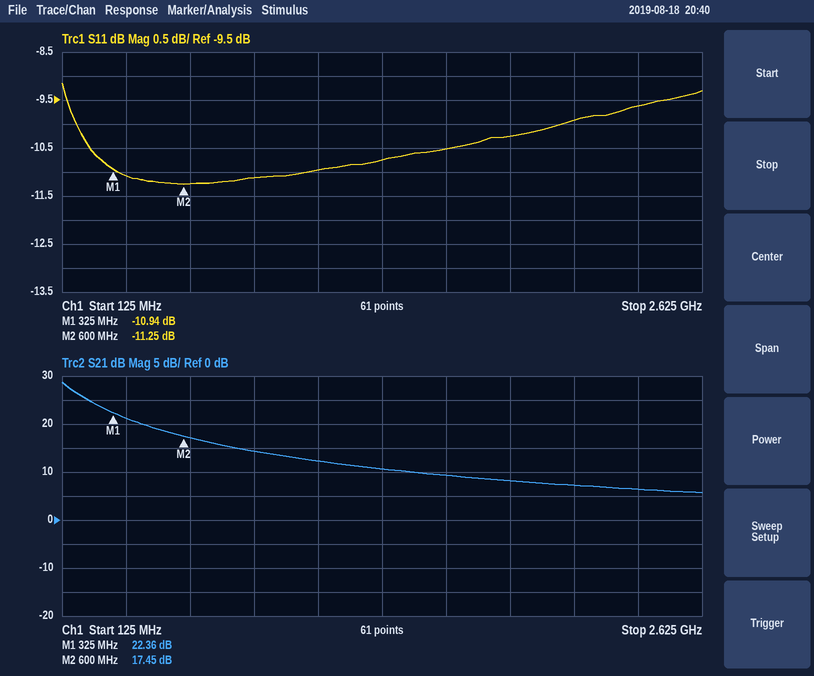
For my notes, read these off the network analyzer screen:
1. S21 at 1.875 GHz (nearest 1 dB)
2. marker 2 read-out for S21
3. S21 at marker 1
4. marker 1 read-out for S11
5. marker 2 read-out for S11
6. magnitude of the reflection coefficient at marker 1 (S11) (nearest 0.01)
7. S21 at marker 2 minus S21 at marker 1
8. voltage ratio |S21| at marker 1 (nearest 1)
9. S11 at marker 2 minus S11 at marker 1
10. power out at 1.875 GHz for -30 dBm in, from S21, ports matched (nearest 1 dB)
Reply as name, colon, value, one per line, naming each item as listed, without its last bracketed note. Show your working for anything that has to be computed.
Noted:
S21 at 1.875 GHz: 8 dB
marker 2 read-out for S21: 17.45 dB
S21 at marker 1: 22.36 dB
marker 1 read-out for S11: -10.94 dB
marker 2 read-out for S11: -11.25 dB
magnitude of the reflection coefficient at marker 1 (S11): 10^(-10.94/20) ≈ 0.28
S21 at marker 2 minus S21 at marker 1: 17.45 − (22.36) = -4.91 dB
voltage ratio |S21| at marker 1: 10^(22.36/20) ≈ 13
S11 at marker 2 minus S11 at marker 1: -11.25 − (-10.94) = -0.31 dB
power out at 1.875 GHz for -30 dBm in, from S21, ports matched: -30 dBm + (8 dB) = -22 dBm
